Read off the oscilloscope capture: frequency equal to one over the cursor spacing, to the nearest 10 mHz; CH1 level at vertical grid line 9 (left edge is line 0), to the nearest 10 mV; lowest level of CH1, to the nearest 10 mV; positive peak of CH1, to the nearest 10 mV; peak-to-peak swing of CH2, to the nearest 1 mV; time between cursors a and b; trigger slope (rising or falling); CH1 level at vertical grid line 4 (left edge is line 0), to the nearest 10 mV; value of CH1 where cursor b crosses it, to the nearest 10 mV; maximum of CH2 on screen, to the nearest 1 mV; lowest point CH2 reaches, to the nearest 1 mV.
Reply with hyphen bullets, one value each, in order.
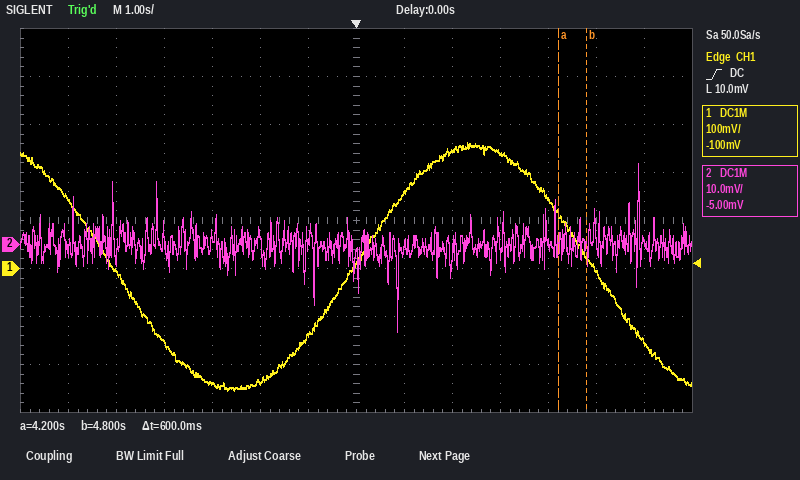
- 1.67 Hz
- 240 mV
- -250 mV
- 260 mV
- 35 mV
- 600 ms
- rising
- -240 mV
- 20 mV
- 17 mV
- -18 mV
